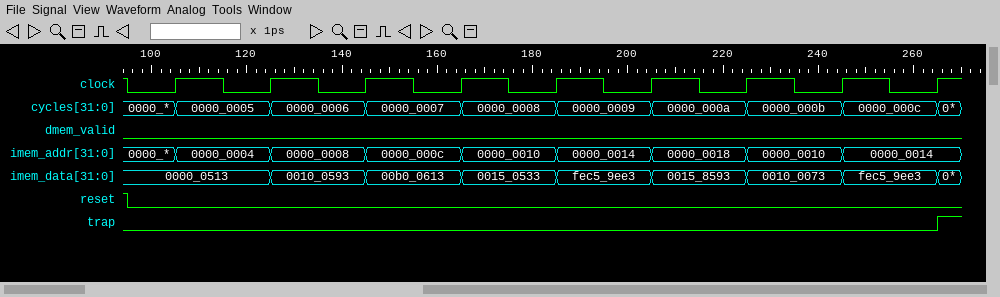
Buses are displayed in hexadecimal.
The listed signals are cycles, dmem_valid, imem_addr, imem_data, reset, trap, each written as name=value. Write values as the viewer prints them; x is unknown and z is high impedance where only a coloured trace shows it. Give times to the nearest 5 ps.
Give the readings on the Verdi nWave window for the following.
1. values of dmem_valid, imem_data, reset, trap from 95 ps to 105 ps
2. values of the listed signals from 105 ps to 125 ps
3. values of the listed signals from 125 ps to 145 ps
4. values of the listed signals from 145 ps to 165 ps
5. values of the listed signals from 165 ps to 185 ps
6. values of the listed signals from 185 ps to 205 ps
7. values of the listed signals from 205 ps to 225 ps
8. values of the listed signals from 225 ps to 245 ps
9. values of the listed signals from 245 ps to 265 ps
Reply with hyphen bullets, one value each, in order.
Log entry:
- dmem_valid=0, imem_data=0000_0513, reset=0, trap=0
- cycles=0000_0005, dmem_valid=0, imem_addr=0000_0004, imem_data=0000_0513, reset=0, trap=0
- cycles=0000_0006, dmem_valid=0, imem_addr=0000_0008, imem_data=0010_0593, reset=0, trap=0
- cycles=0000_0007, dmem_valid=0, imem_addr=0000_000c, imem_data=00b0_0613, reset=0, trap=0
- cycles=0000_0008, dmem_valid=0, imem_addr=0000_0010, imem_data=0015_0533, reset=0, trap=0
- cycles=0000_0009, dmem_valid=0, imem_addr=0000_0014, imem_data=fec5_9ee3, reset=0, trap=0
- cycles=0000_000a, dmem_valid=0, imem_addr=0000_0018, imem_data=0015_8593, reset=0, trap=0
- cycles=0000_000b, dmem_valid=0, imem_addr=0000_0010, imem_data=0010_0073, reset=0, trap=0
- cycles=0000_000c, dmem_valid=0, imem_addr=0000_0014, imem_data=fec5_9ee3, reset=0, trap=0
